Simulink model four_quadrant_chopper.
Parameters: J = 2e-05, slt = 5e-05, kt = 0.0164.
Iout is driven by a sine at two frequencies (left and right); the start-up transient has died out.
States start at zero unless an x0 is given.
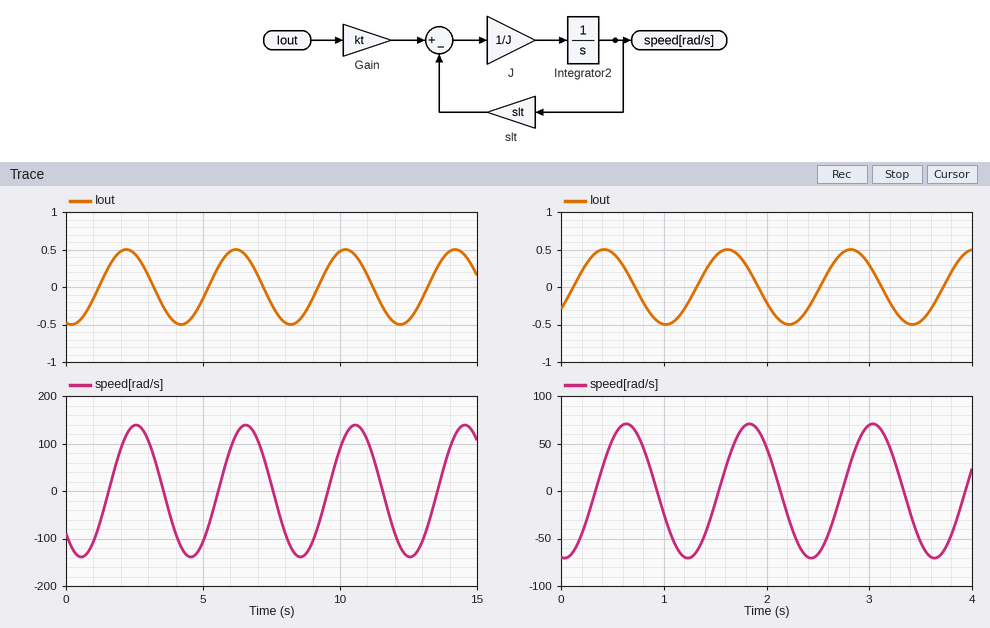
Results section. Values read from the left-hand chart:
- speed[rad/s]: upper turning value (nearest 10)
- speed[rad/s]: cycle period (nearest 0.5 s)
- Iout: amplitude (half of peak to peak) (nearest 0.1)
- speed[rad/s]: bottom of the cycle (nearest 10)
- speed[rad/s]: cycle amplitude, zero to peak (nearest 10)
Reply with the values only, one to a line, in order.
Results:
140
4.0 s
0.5
-140
140
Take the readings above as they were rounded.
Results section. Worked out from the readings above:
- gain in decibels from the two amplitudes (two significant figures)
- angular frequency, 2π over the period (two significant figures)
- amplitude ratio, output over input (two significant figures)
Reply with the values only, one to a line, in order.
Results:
49 dB
1.6 rad/s
280
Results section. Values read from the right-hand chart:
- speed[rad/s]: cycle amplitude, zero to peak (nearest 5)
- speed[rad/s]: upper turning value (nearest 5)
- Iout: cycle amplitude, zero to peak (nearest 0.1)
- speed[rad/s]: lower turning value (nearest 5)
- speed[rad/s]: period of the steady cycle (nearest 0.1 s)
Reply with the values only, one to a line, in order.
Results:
70
70
0.5
-70
1.2 s
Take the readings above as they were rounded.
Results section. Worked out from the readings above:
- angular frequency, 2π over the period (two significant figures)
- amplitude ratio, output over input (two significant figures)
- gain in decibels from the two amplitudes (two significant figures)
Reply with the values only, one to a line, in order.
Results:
5.2 rad/s
140
43 dB
